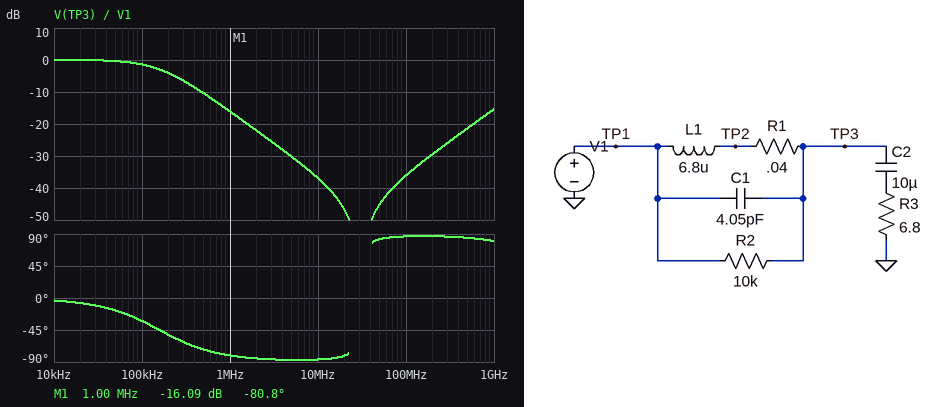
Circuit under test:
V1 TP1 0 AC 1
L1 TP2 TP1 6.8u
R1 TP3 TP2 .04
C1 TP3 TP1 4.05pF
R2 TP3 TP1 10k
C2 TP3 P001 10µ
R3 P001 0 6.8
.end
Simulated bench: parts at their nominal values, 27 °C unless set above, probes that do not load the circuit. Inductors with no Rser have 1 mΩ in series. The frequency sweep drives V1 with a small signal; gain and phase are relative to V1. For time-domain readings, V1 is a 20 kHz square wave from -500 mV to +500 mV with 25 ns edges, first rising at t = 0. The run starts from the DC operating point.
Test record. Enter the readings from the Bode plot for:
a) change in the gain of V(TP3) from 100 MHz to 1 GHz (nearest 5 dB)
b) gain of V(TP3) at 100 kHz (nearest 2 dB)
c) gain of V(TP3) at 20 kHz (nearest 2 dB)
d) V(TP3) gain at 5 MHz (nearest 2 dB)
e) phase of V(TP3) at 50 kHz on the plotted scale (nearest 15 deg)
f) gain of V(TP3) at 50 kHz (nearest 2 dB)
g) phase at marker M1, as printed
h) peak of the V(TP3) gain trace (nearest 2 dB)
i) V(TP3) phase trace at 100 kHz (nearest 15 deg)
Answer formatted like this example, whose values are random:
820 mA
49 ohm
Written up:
20 dB
-2 dB
0 dB
-30 dB
-15 deg
0 dB
-80.8 deg
0 dB
-30 deg
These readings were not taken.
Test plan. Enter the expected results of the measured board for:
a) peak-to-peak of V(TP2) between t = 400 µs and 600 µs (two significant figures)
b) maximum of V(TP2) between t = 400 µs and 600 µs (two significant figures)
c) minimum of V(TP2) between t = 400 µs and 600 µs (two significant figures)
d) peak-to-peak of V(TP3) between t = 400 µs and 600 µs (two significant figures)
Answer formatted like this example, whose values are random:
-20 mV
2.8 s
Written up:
1.0 V
510 mV
-510 mV
1.0 V
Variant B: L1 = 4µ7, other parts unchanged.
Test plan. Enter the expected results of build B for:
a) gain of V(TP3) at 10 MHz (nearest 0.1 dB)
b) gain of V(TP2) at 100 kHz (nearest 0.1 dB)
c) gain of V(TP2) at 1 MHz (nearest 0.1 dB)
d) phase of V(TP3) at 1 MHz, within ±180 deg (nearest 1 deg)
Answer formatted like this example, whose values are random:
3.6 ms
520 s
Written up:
-33.4 dB
-0.7 dB
-12.9 dB
-77 deg
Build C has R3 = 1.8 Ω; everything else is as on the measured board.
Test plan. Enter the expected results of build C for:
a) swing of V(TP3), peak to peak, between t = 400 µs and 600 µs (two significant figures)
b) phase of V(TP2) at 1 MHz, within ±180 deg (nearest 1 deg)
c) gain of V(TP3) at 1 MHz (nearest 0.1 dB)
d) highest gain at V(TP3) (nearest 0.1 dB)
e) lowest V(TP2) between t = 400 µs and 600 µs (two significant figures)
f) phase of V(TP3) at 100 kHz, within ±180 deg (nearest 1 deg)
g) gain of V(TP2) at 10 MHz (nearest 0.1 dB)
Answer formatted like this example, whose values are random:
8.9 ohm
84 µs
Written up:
1.2 V
-88 deg
-27.5 dB
0.9 dB
-590 mV
-71 deg
-48.3 dB
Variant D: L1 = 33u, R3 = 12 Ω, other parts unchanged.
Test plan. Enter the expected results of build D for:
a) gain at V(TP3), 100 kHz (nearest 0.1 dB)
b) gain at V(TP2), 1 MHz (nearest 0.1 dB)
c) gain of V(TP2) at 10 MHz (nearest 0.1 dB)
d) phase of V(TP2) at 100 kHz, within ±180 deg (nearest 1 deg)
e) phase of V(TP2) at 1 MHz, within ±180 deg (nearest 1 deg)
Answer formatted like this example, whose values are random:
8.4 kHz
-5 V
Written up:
-6.0 dB
-24.8 dB
-50.5 dB
-60 deg
-86 deg
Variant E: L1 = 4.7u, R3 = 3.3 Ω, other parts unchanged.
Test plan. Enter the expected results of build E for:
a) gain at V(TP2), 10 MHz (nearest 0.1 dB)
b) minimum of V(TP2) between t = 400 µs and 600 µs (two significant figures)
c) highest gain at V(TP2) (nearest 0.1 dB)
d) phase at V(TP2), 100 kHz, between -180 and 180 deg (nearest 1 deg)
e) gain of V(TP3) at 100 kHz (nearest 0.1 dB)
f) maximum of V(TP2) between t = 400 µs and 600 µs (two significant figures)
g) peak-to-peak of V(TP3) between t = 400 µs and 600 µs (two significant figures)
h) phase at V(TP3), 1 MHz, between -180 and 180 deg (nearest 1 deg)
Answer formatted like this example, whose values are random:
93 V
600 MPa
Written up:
-39.6 dB
-520 mV
0.3 dB
-43 deg
-2.4 dB
520 mV
1.0 V
-84 deg
